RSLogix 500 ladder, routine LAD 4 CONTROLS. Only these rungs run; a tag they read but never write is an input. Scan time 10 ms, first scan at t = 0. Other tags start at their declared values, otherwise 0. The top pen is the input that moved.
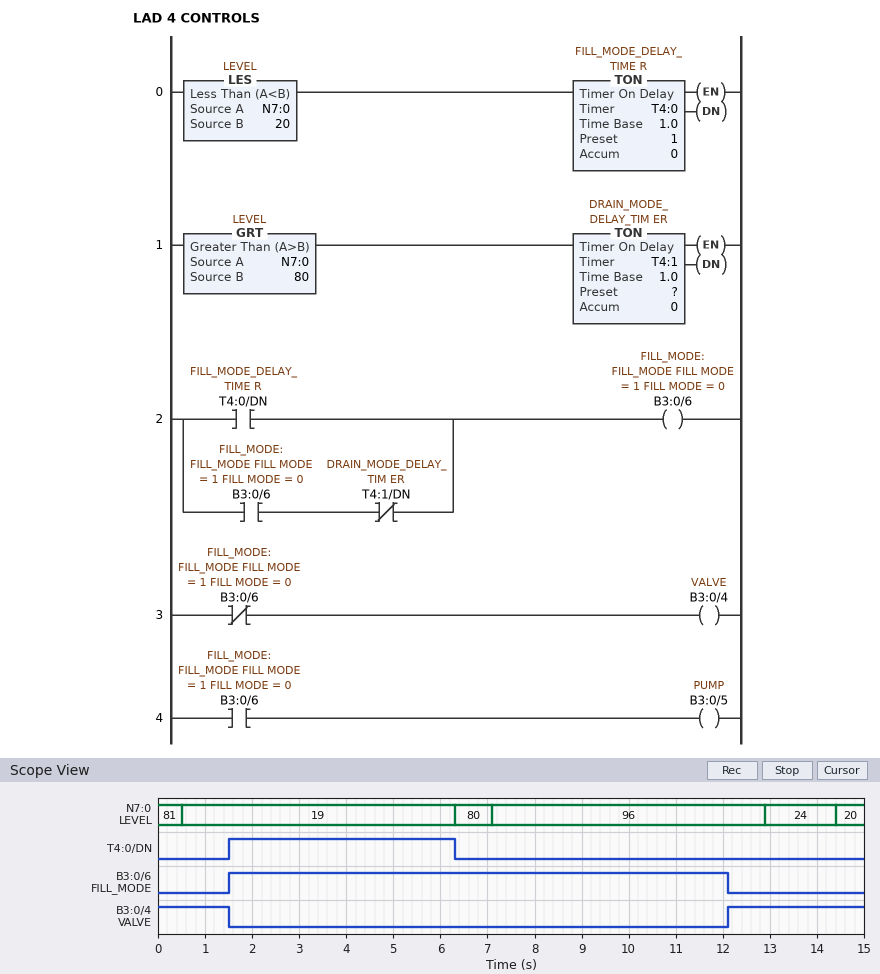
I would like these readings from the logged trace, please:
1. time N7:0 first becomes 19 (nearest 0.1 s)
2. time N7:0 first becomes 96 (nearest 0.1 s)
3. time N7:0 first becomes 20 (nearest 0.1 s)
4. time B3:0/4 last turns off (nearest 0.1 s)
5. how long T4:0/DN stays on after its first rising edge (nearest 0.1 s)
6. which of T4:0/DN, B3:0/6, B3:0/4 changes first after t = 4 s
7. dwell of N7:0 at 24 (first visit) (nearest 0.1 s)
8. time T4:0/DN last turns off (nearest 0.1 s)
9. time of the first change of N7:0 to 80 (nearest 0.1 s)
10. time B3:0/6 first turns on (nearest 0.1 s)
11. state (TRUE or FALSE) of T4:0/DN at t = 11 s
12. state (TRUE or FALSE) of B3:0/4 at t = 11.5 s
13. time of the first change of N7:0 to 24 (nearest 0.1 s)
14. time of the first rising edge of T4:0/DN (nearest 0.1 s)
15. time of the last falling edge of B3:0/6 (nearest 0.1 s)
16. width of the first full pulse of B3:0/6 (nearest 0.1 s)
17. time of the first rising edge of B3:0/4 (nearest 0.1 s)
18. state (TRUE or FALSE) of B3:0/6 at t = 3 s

0.5 s
7.1 s
14.4 s
1.5 s
4.8 s
T4:0/DN
1.5 s
6.3 s
6.3 s
1.5 s
FALSE
FALSE
12.9 s
1.5 s
12.1 s
10.6 s
12.1 s
TRUE
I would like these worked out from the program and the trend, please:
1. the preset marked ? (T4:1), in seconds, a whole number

5 s
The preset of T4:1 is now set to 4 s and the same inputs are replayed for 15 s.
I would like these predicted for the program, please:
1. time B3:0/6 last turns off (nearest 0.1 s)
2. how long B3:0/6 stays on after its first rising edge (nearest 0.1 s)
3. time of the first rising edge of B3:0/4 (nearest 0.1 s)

11.1 s
9.6 s
11.1 s
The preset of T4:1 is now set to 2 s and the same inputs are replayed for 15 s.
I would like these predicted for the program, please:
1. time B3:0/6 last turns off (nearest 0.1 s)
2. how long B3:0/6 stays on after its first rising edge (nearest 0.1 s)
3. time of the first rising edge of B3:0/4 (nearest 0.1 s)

9.1 s
7.6 s
9.1 s
